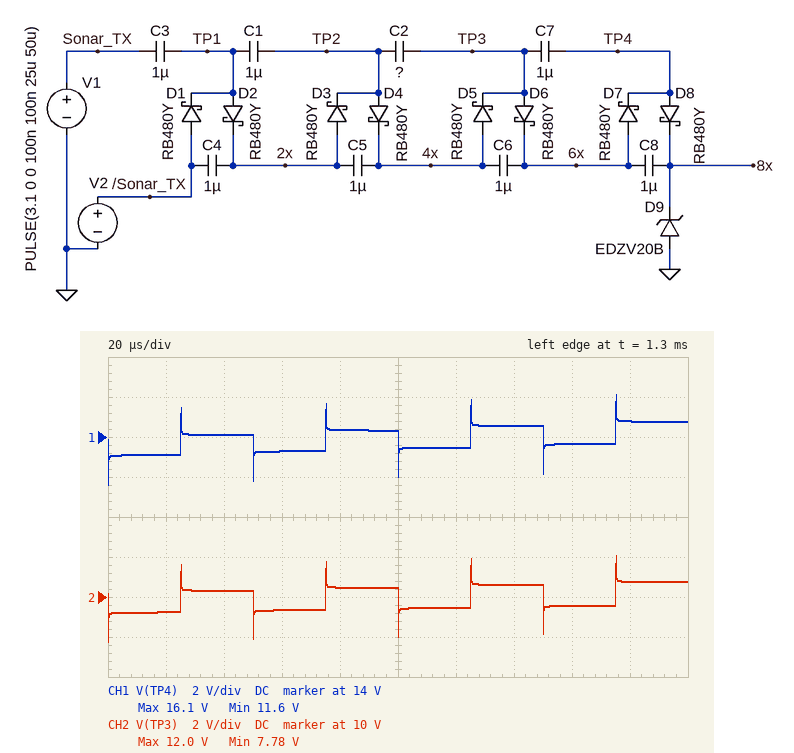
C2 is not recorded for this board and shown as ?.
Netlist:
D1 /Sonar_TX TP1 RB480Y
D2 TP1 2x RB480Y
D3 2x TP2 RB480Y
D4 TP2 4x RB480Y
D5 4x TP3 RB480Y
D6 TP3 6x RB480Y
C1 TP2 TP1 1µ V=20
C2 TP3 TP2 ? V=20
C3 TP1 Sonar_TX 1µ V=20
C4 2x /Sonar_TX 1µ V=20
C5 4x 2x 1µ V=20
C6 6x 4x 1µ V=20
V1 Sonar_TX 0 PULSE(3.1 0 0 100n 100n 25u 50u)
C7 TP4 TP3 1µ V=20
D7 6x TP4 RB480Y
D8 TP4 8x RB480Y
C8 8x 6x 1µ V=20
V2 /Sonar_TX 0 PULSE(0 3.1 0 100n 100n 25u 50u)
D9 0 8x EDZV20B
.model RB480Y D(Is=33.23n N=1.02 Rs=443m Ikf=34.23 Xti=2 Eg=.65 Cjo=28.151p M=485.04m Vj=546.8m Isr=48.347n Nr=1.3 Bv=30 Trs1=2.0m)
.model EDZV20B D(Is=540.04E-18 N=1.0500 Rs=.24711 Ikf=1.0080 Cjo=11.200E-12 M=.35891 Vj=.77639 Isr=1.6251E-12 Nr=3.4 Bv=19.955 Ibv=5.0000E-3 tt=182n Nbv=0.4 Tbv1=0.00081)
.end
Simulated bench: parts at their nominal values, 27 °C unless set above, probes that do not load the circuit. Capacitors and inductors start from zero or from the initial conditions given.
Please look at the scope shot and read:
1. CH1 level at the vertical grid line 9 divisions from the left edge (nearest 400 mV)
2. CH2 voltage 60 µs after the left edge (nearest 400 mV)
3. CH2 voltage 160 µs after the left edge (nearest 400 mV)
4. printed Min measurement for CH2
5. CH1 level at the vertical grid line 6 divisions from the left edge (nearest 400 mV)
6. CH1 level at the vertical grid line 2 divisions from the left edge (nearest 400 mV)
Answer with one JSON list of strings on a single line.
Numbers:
["14.8 V", "9.2 V", "9.6 V", "7.78 V", "13.6 V", "14.0 V"]
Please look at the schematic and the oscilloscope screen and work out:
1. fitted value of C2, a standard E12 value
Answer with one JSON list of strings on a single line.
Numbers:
["10 µF"]
